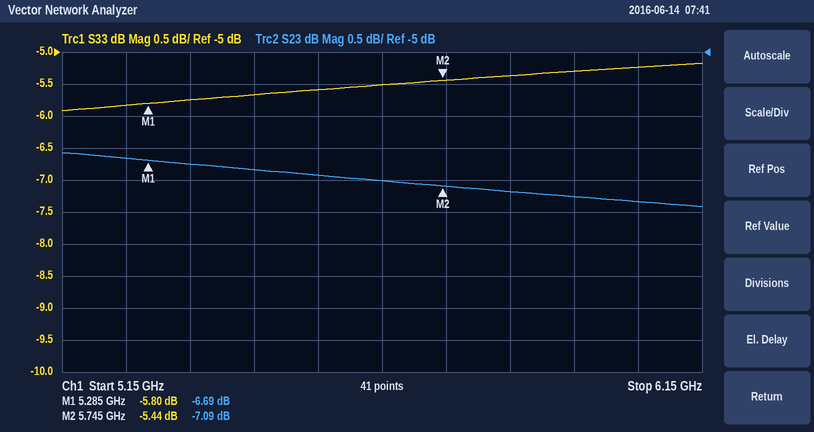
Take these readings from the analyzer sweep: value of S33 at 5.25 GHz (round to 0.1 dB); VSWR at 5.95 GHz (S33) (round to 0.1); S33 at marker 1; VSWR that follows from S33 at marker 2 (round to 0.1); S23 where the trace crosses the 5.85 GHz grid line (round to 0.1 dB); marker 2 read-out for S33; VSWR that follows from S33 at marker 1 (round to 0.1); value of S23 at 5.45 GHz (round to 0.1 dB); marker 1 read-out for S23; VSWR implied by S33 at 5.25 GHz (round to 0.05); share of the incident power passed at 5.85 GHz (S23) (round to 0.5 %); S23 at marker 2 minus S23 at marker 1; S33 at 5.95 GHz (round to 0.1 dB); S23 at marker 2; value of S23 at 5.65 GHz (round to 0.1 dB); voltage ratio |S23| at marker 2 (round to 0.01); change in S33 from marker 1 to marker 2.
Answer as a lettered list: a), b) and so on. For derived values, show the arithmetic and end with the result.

a) -5.8 dB
b) |Γ| = 10^(-5.3/20) = 0.5433; VSWR = (1 + 0.5433)/(1 − 0.5433) ≈ 3.4
c) -5.80 dB
d) (1 + 0.5346)/(1 − 0.5346) ≈ 3.3
e) -7.2 dB
f) -5.44 dB
g) (1 + 0.5129)/(1 − 0.5129) ≈ 3.1
h) -6.8 dB
i) -6.69 dB
j) |Γ| = 10^(-5.8/20) = 0.5129; VSWR = (1 + 0.5129)/(1 − 0.5129) ≈ 3.11, so 3.10 to the nearest 0.05
k) 10^(-7.2/10) ≈ 19.1 %, so 19.0 % to the nearest 0.5 %
l) -7.09 − (-6.69) = -0.40 dB
m) -5.3 dB
n) -7.09 dB
o) -7.0 dB
p) 10^(-7.09/20) ≈ 0.44
q) -5.44 − (-5.8) = 0.36 dB
